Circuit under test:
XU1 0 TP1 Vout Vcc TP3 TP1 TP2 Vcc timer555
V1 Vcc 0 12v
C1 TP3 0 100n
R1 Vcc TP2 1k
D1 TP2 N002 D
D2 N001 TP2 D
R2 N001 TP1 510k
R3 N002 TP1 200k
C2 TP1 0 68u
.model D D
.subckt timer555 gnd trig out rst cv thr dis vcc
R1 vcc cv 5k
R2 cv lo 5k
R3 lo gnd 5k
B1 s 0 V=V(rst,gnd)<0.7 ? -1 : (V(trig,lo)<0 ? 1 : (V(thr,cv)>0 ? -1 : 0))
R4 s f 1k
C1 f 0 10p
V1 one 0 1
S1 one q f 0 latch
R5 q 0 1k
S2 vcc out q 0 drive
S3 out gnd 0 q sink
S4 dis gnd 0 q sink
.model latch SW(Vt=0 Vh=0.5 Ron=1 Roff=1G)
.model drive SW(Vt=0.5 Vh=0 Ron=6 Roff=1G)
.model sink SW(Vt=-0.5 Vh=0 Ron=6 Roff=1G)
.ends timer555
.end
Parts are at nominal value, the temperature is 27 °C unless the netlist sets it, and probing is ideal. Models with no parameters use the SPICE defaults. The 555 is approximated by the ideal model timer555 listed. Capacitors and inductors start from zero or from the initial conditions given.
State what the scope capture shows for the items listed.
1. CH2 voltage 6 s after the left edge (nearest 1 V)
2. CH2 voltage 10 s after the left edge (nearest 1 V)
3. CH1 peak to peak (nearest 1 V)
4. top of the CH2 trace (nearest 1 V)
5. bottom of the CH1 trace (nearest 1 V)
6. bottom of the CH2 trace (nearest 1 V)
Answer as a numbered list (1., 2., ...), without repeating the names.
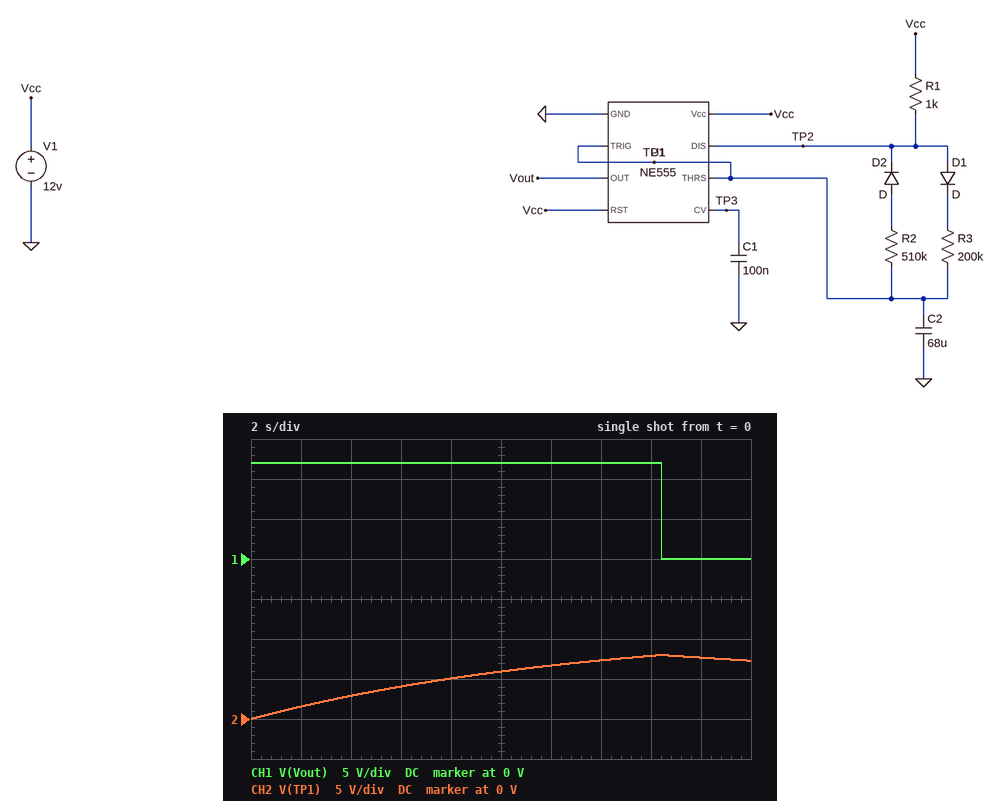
1. 4 V
2. 6 V
3. 12 V
4. 8 V
5. 0 V
6. 0 V
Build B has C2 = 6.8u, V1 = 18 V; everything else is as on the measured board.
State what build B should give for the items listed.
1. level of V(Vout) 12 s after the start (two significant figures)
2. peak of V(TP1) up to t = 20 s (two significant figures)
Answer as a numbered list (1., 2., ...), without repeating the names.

1. 18 V
2. 12 V
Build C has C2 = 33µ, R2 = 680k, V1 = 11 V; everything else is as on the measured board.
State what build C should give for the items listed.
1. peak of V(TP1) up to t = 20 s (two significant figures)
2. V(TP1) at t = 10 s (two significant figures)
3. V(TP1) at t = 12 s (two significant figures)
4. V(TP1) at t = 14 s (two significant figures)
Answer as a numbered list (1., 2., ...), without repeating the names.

1. 7.3 V
2. 6.8 V
3. 6.2 V
4. 5.8 V
